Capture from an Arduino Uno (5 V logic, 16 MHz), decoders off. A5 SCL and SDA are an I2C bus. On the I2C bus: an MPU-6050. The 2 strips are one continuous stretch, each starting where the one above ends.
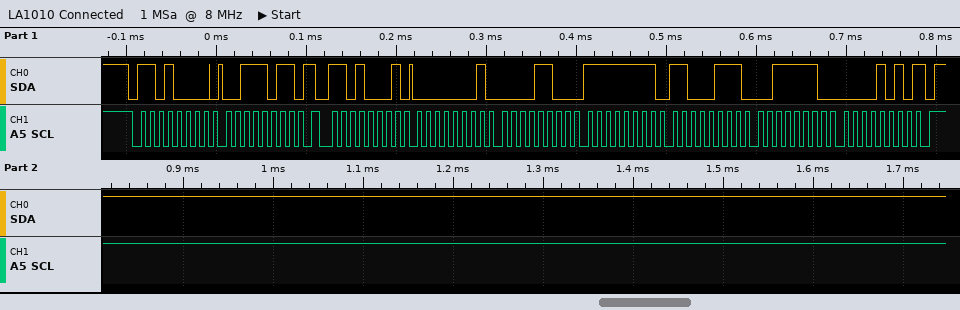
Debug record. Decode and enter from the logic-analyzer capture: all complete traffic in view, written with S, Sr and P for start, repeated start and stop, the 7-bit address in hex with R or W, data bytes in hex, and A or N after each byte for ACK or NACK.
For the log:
S 68W A 3B A Sr 68R A 01 A 0C A FF A C7 A 3E A 0A N P
